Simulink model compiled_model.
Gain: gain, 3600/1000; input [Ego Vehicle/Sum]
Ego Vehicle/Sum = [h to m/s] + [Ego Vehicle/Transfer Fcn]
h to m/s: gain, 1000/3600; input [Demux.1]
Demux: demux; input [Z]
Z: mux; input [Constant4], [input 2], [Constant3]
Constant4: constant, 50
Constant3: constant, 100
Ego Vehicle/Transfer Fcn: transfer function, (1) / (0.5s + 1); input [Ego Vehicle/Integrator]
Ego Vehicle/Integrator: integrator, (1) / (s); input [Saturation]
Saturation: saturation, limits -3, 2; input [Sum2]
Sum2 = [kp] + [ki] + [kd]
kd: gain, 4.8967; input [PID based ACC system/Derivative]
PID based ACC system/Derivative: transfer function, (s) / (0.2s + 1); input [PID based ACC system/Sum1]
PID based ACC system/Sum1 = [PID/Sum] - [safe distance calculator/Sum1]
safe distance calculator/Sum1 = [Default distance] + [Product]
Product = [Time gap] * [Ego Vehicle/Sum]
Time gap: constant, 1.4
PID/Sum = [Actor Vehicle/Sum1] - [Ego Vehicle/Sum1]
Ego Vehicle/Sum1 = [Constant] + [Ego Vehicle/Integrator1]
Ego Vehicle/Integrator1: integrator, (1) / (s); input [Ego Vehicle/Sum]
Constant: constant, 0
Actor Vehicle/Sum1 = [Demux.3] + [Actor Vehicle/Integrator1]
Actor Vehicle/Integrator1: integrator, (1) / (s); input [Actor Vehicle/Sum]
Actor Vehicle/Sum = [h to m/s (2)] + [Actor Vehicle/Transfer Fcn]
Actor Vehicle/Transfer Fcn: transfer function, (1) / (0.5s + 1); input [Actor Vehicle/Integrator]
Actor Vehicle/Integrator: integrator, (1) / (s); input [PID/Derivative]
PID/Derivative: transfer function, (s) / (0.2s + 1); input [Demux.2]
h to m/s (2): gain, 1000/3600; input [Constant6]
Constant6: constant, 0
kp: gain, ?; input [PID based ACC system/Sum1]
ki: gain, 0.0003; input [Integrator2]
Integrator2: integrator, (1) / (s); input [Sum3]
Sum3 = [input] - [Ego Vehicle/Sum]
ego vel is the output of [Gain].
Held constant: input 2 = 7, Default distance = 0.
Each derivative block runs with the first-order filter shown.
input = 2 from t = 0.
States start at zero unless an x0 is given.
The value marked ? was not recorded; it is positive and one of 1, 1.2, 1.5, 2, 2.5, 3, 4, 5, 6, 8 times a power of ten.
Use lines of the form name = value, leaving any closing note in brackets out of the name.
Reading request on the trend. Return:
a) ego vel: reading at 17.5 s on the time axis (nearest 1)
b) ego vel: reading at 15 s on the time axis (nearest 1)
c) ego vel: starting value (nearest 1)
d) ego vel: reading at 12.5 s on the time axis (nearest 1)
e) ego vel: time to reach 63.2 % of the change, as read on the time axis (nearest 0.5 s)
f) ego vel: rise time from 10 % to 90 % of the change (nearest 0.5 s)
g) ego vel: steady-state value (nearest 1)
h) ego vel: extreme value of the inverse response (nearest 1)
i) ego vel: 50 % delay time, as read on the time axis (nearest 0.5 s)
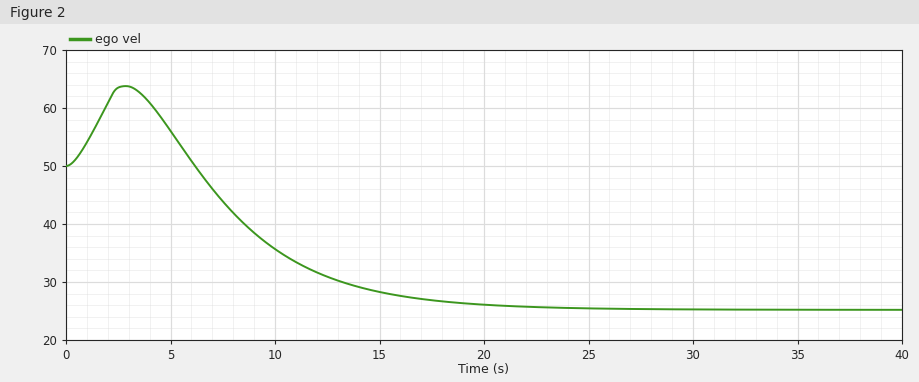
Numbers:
ego vel: reading at 17.5 s on the time axis = 27
ego vel: reading at 15 s on the time axis = 28
ego vel: starting value = 50
ego vel: reading at 12.5 s on the time axis = 31
ego vel: time to reach 63.2 % of the change, as read on the time axis = 10.5 s
ego vel: rise time from 10 % to 90 % of the change = 9.0 s
ego vel: steady-state value = 25
ego vel: extreme value of the inverse response = 64
ego vel: 50 % delay time, as read on the time axis = 9.5 s
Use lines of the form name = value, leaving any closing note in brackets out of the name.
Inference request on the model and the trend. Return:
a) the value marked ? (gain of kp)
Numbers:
the value marked ? = 1.2
